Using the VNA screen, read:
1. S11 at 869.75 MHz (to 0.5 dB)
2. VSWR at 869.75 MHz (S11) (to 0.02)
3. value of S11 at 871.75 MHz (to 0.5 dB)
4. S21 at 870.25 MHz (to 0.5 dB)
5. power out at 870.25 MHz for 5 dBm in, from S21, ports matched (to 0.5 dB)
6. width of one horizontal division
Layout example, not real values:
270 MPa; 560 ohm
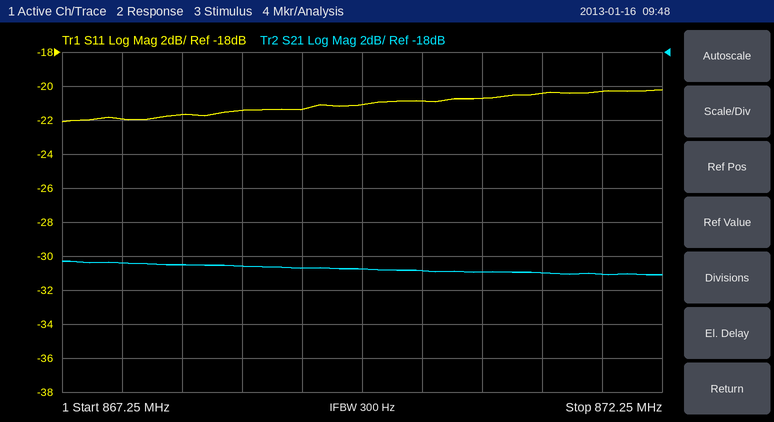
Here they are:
-21.0 dB; 1.20; -20.5 dB; -31.0 dB; -26.0 dBm; 500 kHz
